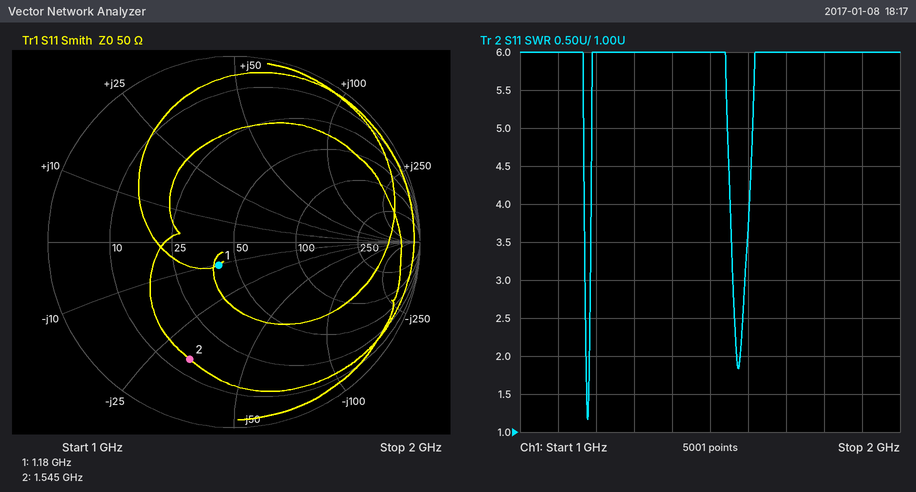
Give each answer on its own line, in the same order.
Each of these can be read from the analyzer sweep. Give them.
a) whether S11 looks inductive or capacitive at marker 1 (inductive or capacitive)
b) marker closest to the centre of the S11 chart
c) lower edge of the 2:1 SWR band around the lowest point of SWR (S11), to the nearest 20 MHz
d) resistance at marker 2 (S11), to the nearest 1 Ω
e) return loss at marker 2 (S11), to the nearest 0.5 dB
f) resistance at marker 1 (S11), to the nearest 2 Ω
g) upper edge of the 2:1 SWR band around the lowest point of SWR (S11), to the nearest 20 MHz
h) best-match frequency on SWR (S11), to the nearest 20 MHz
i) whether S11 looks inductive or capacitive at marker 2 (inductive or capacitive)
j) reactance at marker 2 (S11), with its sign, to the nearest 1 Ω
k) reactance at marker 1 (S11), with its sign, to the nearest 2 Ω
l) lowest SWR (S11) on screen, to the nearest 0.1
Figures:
capacitive
marker 1
1.18 GHz
14 Ω
3.5 dB
42 Ω
1.18 GHz
1.18 GHz
capacitive
-33 Ω
-10 Ω
1.2
